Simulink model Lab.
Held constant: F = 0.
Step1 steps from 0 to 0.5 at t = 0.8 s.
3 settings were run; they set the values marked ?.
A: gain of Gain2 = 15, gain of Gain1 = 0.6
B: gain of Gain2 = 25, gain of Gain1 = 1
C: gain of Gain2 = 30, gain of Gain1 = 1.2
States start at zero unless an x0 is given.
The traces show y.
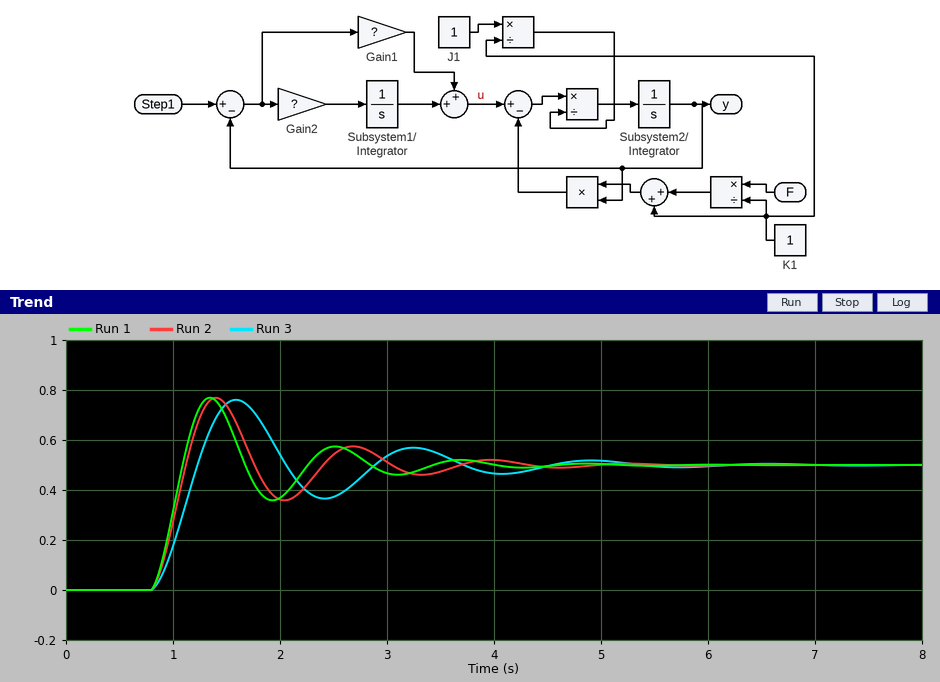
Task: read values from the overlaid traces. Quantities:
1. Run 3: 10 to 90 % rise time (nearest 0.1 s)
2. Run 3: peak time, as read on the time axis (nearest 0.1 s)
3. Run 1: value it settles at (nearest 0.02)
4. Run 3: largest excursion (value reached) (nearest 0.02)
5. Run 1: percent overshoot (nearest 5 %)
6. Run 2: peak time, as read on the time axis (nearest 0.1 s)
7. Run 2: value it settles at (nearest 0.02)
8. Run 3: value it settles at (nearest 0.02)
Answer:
0.3 s
1.6 s
0.50
0.76
55 %
1.4 s
0.50
0.50
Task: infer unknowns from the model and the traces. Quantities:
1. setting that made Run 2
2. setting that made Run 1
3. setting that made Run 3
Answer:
B
C
A
